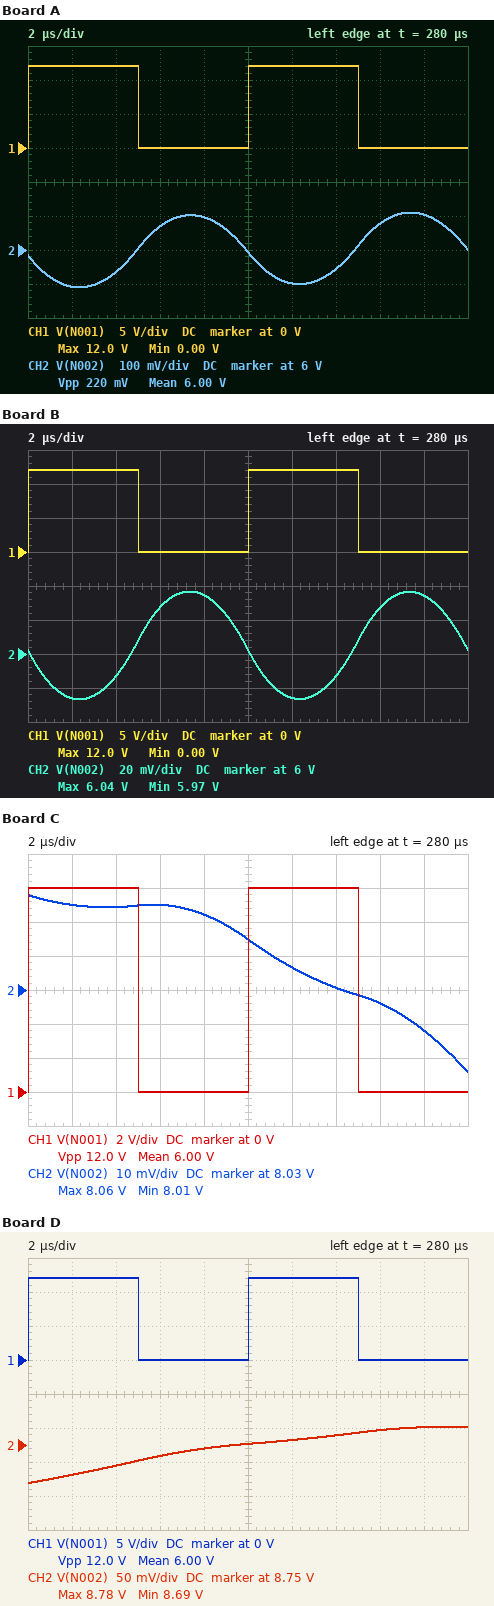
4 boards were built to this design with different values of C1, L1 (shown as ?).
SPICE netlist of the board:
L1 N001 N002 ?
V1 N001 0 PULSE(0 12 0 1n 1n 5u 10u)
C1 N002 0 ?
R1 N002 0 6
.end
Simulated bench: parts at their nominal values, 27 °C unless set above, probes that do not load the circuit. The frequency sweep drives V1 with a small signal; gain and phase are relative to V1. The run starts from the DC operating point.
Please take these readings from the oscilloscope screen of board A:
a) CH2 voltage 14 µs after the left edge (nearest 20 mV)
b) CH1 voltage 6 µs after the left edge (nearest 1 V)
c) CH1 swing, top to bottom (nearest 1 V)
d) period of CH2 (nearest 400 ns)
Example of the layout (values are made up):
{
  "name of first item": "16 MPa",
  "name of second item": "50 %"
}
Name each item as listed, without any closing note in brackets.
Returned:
{
  "CH2 voltage 14 µs after the left edge": "5.94 V",
  "CH1 voltage 6 µs after the left edge": "0 V",
  "CH1 swing, top to bottom": "12 V",
  "period of CH2": "10.0 µs"
}
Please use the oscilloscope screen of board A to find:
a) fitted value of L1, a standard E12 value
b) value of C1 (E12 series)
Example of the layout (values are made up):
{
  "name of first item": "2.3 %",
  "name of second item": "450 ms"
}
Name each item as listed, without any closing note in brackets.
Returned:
{
  "fitted value of L1, a standard E12 value": "47 µH",
  "value of C1": "3.9 µF"
}
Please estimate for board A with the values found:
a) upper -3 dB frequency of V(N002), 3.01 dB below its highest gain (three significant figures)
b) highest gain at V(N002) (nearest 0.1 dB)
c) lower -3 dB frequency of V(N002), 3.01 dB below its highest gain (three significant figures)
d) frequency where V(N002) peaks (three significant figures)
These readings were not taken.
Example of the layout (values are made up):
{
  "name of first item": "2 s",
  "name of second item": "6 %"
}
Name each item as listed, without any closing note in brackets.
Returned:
{
  "upper -3 dB frequency of V(N002), 3.01 dB below its highest gain": "13.8 kHz",
  "highest gain at V(N002)": "5.1 dB",
  "lower -3 dB frequency of V(N002), 3.01 dB below its highest gain": "6.21 kHz",
  "frequency where V(N002) peaks": "10.7 kHz"
}
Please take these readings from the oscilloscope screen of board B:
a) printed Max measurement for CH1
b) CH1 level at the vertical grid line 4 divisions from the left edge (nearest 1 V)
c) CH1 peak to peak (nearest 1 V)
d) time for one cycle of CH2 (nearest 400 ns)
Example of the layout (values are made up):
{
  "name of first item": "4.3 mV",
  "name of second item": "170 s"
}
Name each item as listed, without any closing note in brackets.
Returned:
{
  "printed Max measurement for CH1": "12.0 V",
  "CH1 level at the vertical grid line 4 divisions from the left edge": "0 V",
  "CH1 peak to peak": "12 V",
  "time for one cycle of CH2": "10.0 µs"
}
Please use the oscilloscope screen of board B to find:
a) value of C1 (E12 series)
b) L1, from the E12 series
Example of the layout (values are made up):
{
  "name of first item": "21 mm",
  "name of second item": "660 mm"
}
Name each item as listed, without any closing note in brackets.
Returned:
{
  "value of C1": "3.3 µF",
  "L1, from the E12 series": "180 µH"
}
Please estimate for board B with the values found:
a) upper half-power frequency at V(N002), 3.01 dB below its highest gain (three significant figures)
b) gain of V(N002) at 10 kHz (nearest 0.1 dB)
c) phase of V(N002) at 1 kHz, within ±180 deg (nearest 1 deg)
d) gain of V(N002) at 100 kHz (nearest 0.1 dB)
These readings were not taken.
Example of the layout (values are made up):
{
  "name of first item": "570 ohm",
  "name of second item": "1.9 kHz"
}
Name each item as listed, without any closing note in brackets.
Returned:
{
  "upper half-power frequency at V(N002), 3.01 dB below its highest gain": "7.19 kHz",
  "gain of V(N002) at 10 kHz": "-7.3 dB",
  "phase of V(N002) at 1 kHz, within ±180 deg": "-11 deg",
  "gain of V(N002) at 100 kHz": "-47.4 dB"
}
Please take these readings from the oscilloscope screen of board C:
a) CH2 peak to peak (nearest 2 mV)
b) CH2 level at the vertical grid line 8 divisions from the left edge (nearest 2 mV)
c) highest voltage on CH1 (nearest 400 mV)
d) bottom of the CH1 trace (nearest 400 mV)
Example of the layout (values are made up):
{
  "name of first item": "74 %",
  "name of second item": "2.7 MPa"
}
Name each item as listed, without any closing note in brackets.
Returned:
{
  "CH2 peak to peak": "52 mV",
  "CH2 level at the vertical grid line 8 divisions from the left edge": "8.026 V",
  "highest voltage on CH1": "12.0 V",
  "bottom of the CH1 trace": "0 V"
}
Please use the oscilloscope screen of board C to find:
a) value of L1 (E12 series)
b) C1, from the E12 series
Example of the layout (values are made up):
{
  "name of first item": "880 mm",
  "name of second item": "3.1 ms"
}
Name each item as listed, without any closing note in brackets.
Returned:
{
  "value of L1": "330 µH",
  "C1, from the E12 series": "22 µF"
}
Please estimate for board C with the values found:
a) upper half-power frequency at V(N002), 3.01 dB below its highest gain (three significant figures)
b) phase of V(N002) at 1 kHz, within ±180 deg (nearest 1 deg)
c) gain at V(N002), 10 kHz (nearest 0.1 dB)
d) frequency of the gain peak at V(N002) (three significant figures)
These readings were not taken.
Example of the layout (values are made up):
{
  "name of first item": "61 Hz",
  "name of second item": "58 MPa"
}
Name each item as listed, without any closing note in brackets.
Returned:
{
  "upper half-power frequency at V(N002), 3.01 dB below its highest gain": "2.21 kHz",
  "phase of V(N002) at 1 kHz, within ±180 deg": "-26 deg",
  "gain at V(N002), 10 kHz": "-28.9 dB",
  "frequency of the gain peak at V(N002)": "1.66 kHz"
}
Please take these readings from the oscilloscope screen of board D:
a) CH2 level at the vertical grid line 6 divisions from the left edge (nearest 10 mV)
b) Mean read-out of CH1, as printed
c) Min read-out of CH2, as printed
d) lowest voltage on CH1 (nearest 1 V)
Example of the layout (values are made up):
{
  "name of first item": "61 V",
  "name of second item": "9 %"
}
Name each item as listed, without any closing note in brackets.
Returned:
{
  "CH2 level at the vertical grid line 6 divisions from the left edge": "8.76 V",
  "Mean read-out of CH1, as printed": "6.00 V",
  "Min read-out of CH2, as printed": "8.69 V",
  "lowest voltage on CH1": "0 V"
}
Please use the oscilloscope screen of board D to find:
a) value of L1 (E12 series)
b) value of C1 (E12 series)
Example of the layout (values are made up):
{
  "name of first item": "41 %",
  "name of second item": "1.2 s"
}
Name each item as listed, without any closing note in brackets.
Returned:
{
  "value of L1": "270 µH",
  "value of C1": "33 µF"
}
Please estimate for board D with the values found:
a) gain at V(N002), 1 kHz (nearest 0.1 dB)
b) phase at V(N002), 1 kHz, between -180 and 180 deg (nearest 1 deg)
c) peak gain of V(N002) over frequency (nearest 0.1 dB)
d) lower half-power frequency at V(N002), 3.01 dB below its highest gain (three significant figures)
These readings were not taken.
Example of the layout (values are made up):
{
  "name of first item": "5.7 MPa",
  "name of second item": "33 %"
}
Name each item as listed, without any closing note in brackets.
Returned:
{
  "gain at V(N002), 1 kHz": "3.0 dB",
  "phase at V(N002), 1 kHz, between -180 and 180 deg": "-24 deg",
  "peak gain of V(N002) over frequency": "6.7 dB",
  "lower half-power frequency at V(N002), 3.01 dB below its highest gain": "1.10 kHz"
}
